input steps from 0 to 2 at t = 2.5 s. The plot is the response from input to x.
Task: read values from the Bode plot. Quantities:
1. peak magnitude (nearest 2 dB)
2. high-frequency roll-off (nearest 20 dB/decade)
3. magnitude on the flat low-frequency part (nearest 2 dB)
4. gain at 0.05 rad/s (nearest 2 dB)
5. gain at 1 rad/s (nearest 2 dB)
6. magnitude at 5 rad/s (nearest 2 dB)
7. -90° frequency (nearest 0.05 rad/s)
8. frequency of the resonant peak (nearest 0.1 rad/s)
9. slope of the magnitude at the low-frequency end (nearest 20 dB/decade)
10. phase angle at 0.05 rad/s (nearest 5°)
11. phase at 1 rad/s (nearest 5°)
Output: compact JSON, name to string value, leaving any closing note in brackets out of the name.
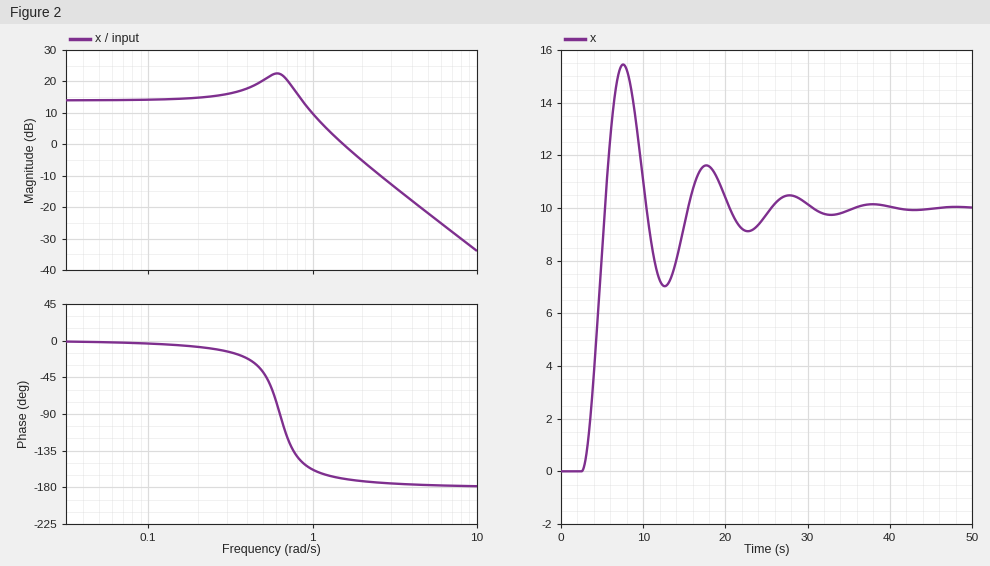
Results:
{"peak magnitude": "22 dB", "high-frequency roll-off": "-40 dB/decade", "magnitude on the flat low-frequency part": "14 dB", "gain at 0.05 rad/s": "14 dB", "gain at 1 rad/s": "10 dB", "magnitude at 5 rad/s": "-22 dB", "-90° frequency": "0.65 rad/s", "frequency of the resonant peak": "0.6 rad/s", "slope of the magnitude at the low-frequency end": "0 dB/decade", "phase angle at 0.05 rad/s": "0°", "phase at 1 rad/s": "-160°"}
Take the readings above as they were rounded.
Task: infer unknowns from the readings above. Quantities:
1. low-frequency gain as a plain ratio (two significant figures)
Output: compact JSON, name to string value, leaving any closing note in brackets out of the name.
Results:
{"low-frequency gain as a plain ratio": "5.0"}
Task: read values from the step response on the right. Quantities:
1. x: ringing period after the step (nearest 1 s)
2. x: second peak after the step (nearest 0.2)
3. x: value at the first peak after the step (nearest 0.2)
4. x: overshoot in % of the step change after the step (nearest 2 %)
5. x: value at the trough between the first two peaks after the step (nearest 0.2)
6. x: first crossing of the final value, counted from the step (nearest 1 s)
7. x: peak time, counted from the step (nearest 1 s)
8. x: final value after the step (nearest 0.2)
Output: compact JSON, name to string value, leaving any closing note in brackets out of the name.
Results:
{"x: ringing period after the step": "10 s", "x: second peak after the step": "11.6", "x: value at the first peak after the step": "15.4", "x: overshoot in % of the step change after the step": "54 %", "x: value at the trough between the first two peaks after the step": "7.0", "x: first crossing of the final value, counted from the step": "3 s", "x: peak time, counted from the step": "5 s", "x: final value after the step": "10.0"}
